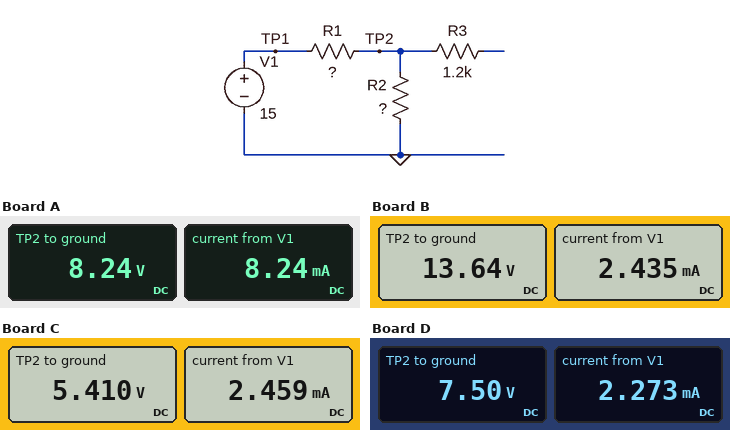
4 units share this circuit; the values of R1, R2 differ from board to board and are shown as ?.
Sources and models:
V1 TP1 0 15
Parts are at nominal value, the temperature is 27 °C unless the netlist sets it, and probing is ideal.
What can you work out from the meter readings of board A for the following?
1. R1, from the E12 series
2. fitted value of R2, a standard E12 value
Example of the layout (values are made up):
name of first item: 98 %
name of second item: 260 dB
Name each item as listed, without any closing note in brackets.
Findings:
R1, from the E12 series: 820 Ω
fitted value of R2, a standard E12 value: 1 kΩ
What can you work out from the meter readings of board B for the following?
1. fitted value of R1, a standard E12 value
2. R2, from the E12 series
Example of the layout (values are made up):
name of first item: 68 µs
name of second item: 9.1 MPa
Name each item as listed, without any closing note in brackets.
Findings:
fitted value of R1, a standard E12 value: 560 Ω
R2, from the E12 series: 5.6 kΩ
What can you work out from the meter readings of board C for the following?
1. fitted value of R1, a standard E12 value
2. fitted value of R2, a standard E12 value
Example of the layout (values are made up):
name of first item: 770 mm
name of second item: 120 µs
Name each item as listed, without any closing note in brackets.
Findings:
fitted value of R1, a standard E12 value: 3.9 kΩ
fitted value of R2, a standard E12 value: 2.2 kΩ
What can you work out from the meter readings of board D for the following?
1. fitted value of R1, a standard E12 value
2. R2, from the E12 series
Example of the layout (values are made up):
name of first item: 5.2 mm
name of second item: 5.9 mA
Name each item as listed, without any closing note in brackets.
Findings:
fitted value of R1, a standard E12 value: 3.3 kΩ
R2, from the E12 series: 3.3 kΩ
